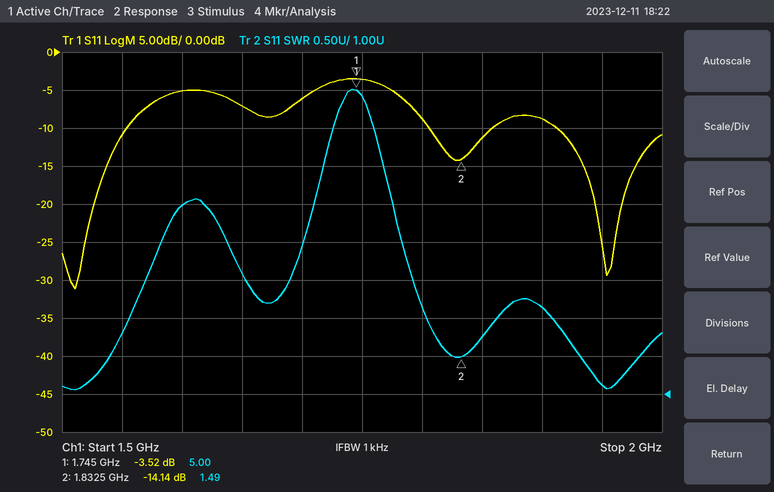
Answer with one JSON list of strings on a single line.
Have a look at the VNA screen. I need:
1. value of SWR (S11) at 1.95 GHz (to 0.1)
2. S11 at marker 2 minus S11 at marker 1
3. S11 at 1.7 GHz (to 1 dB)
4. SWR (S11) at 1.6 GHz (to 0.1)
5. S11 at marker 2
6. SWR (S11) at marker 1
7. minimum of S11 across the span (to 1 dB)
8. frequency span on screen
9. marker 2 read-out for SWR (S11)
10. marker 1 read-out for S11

["1.1", "-10.62 dB", "-6 dB", "3.5", "-14.14 dB", "5.00", "-31 dB", "500 MHz", "1.49", "-3.52 dB"]
